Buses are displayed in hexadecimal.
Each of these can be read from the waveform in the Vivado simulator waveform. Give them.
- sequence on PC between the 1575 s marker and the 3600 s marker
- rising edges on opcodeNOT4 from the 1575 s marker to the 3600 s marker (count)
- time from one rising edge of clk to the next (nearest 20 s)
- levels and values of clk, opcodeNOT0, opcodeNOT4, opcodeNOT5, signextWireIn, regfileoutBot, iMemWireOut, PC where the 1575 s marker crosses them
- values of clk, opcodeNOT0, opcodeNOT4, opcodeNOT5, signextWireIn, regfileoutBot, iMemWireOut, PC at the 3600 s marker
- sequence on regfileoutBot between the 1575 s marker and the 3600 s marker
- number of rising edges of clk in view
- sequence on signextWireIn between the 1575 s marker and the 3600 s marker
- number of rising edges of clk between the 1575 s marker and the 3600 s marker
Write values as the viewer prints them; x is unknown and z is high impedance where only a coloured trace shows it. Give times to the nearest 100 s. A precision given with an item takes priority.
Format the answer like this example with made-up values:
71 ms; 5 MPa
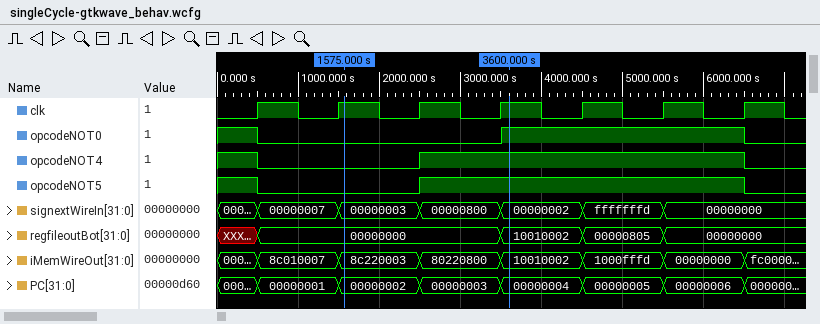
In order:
00000002, 00000003, 00000004; 1; 1000 s; clk=1, opcodeNOT0=0, opcodeNOT4=0, opcodeNOT5=0, signextWireIn=00000003, regfileoutBot=00000000, iMemWireOut=8c220003, PC=00000002; clk=1, opcodeNOT0=1, opcodeNOT4=1, opcodeNOT5=1, signextWireIn=00000002, regfileoutBot=10010002, iMemWireOut=10010002, PC=00000004; 00000000, 10010002; 7; 00000003, 00000800, 00000002; 2
